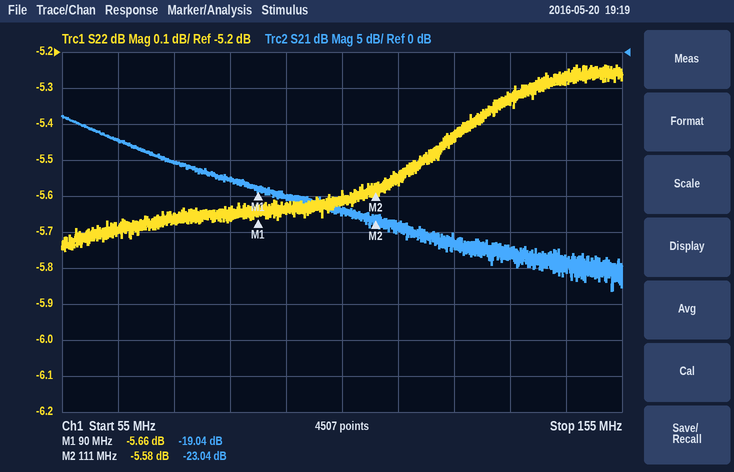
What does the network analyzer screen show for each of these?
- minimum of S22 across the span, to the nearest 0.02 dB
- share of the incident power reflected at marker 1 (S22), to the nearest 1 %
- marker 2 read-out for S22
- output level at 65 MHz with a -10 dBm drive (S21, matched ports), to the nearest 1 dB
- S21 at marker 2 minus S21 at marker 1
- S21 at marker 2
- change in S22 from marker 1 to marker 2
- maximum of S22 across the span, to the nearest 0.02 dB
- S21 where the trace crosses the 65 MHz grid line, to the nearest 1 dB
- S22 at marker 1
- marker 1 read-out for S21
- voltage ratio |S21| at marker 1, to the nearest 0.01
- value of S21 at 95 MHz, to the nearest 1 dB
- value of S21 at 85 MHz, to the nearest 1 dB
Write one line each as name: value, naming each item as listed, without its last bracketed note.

minimum of S22 across the span, to the nearest 0.02 dB: -5.76 dB
share of the incident power reflected at marker 1 (S22), to the nearest 1 %: 27 %
marker 2 read-out for S22: -5.58 dB
output level at 65 MHz with a -10 dBm drive (S21, matched ports), to the nearest 1 dB: -22 dBm
S21 at marker 2 minus S21 at marker 1: -4.00 dB
S21 at marker 2: -23.04 dB
change in S22 from marker 1 to marker 2: 0.08 dB
maximum of S22 across the span, to the nearest 0.02 dB: -5.24 dB
S21 where the trace crosses the 65 MHz grid line, to the nearest 1 dB: -12 dB
S22 at marker 1: -5.66 dB
marker 1 read-out for S21: -19.04 dB
voltage ratio |S21| at marker 1, to the nearest 0.01: 0.11
value of S21 at 95 MHz, to the nearest 1 dB: -20 dB
value of S21 at 85 MHz, to the nearest 1 dB: -18 dB
